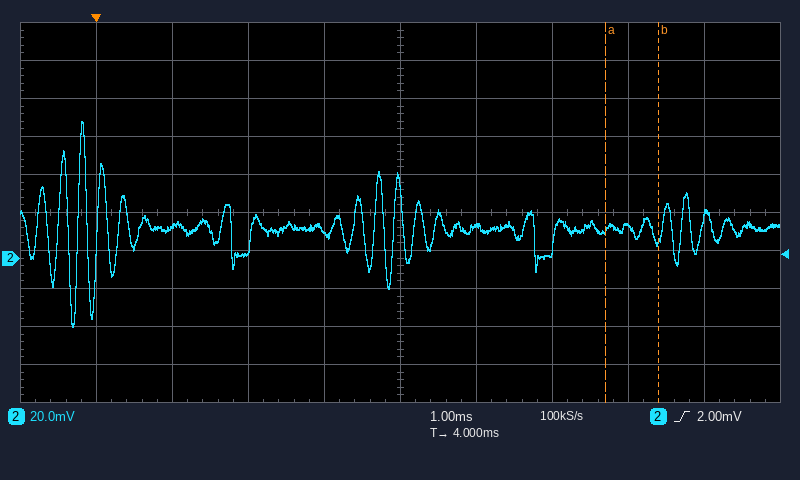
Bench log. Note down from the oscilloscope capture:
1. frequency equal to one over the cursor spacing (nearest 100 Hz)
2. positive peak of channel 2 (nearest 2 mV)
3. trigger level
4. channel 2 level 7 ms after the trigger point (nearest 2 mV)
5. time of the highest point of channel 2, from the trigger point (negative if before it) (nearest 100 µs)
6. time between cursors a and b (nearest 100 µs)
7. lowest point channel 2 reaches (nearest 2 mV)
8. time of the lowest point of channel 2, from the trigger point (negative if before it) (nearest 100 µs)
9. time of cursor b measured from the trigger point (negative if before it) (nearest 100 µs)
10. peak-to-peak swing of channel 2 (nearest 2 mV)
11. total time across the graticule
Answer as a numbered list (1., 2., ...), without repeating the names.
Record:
1. 1.4 kHz
2. 72 mV
3. 2.00 mV
4. 16 mV
5. -200 µs
6. 700 µs
7. -36 mV
8. -300 µs
9. +7.4 ms
10. 108 mV
11. 10 ms
